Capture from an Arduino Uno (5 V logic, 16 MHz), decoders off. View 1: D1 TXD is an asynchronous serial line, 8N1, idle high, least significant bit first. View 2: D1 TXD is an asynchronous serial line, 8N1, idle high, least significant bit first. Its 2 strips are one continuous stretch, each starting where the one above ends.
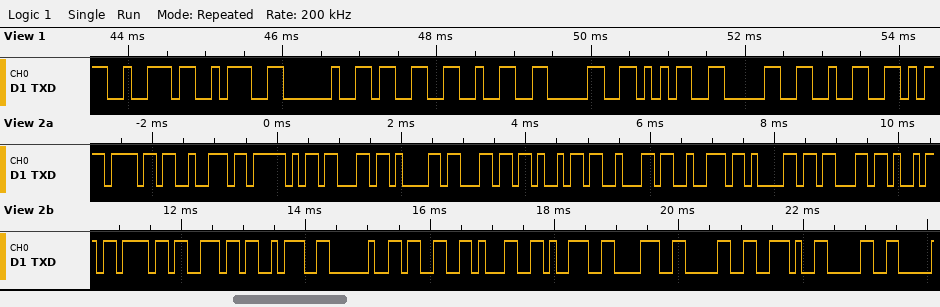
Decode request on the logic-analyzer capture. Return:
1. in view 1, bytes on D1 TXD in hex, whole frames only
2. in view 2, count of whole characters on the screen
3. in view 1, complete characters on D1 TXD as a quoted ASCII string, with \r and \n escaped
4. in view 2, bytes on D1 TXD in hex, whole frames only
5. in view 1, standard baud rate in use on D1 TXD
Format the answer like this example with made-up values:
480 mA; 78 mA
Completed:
72 3A 20 33 32 30 35 30 32; 23; "r: 320502"; 6F 72 5F 63 61 6C 69 62 72 61 63 69 6F 6E 3A 20 33 31 39 38 30 2E 30; 9600 baud
